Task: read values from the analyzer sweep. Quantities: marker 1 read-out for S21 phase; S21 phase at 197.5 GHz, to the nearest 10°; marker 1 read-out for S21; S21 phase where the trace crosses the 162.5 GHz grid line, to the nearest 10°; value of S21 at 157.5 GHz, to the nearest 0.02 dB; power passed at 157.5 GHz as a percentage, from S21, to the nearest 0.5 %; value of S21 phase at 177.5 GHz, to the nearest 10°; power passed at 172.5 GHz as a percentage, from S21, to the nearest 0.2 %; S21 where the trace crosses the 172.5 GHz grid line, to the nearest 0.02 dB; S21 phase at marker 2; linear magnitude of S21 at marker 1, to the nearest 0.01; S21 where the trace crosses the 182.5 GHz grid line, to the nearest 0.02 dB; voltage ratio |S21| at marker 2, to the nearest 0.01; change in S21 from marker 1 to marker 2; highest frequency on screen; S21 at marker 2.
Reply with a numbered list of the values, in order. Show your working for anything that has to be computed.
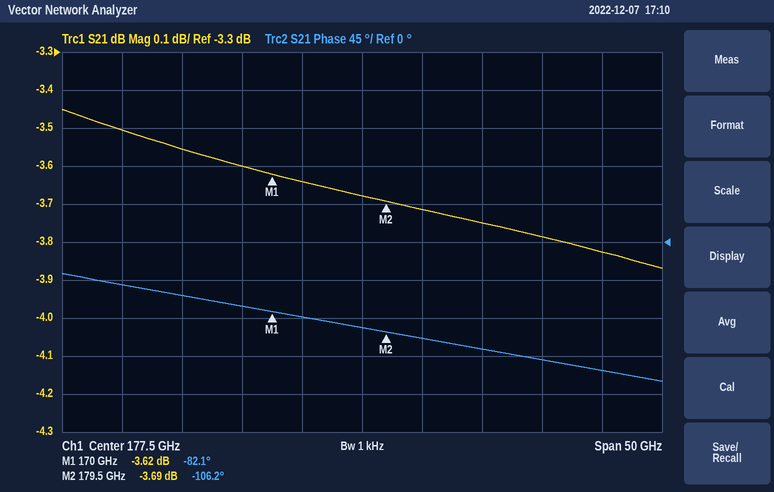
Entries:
1. -82.1°
2. -150°
3. -3.62 dB
4. -60°
5. -3.50 dB
6. 10^(-3.5/10) ≈ 44.7 %, so 44.5 % to the nearest 0.5 %
7. -100°
8. 10^(-3.64/10) ≈ 43.3 %, so 43.2 % to the nearest 0.2 %
9. -3.64 dB
10. -106.2°
11. 10^(-3.62/20) ≈ 0.66
12. -3.72 dB
13. 10^(-3.69/20) ≈ 0.65
14. -3.69 − (-3.62) = -0.07 dB
15. 202.5 GHz
16. -3.69 dB
